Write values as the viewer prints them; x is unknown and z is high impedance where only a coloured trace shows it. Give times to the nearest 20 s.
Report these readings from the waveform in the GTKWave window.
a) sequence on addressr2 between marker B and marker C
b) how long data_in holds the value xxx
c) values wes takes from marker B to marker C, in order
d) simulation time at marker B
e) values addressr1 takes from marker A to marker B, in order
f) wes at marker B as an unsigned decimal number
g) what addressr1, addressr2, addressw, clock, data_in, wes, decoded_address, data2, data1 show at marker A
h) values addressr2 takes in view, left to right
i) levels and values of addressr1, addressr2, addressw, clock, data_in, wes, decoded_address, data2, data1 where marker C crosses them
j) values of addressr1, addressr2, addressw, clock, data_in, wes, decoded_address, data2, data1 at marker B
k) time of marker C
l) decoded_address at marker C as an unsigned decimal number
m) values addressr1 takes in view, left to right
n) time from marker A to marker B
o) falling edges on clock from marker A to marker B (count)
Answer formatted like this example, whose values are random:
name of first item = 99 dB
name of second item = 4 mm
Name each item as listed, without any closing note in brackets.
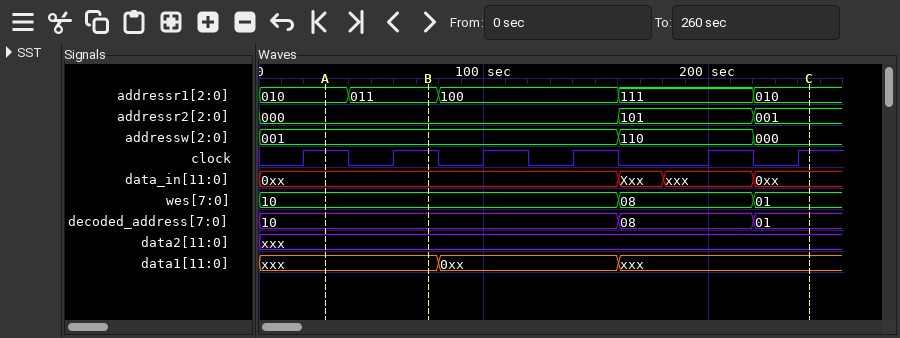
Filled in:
sequence on addressr2 between marker B and marker C = 000, 101, 001
how long data_in holds the value xxx = 40 s
values wes takes from marker B to marker C, in order = 10, 08, 01
simulation time at marker B = 80 s
values addressr1 takes from marker A to marker B, in order = 010, 011
wes at marker B as an unsigned decimal number = 16
what addressr1, addressr2, addressw, clock, data_in, wes, decoded_address, data2, data1 show at marker A = addressr1=010, addressr2=000, addressw=001, clock=1, data_in=0xx, wes=10, decoded_address=10, data2=xxx, data1=xxx
values addressr2 takes in view, left to right = 000, 101, 001
levels and values of addressr1, addressr2, addressw, clock, data_in, wes, decoded_address, data2, data1 where marker C crosses them = addressr1=010, addressr2=001, addressw=000, clock=1, data_in=0xx, wes=01, decoded_address=01, data2=xxx, data1=xxx
values of addressr1, addressr2, addressw, clock, data_in, wes, decoded_address, data2, data1 at marker B = addressr1=011, addressr2=000, addressw=001, clock=1, data_in=0xx, wes=10, decoded_address=10, data2=xxx, data1=xxx
time of marker C = 240 s
decoded_address at marker C as an unsigned decimal number = 1
values addressr1 takes in view, left to right = 010, 011, 100, 111, 010
time from marker A to marker B = 40 s
falling edges on clock from marker A to marker B = 1
